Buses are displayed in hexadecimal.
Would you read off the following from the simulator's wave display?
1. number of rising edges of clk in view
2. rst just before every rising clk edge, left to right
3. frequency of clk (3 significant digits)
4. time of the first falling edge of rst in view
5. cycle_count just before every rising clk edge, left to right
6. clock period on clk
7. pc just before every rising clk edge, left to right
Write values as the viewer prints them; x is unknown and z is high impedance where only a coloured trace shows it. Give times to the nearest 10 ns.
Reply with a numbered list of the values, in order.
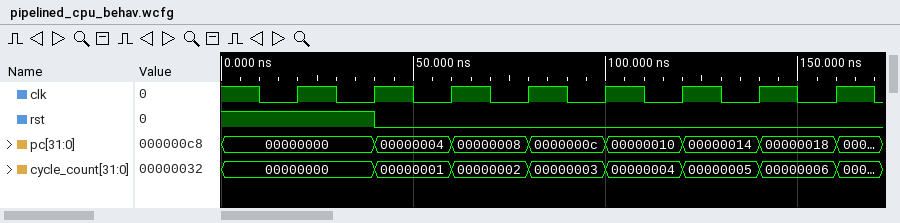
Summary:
1. 8
2. 1 1 0 0 0 0 0 0
3. 50.0 MHz
4. 40 ns
5. 00000000, 00000000, 00000001, 00000002, 00000003, 00000004, 00000005, 00000006
6. 20 ns
7. 00000000, 00000000, 00000004, 00000008, 0000000c, 00000010, 00000014, 00000018
